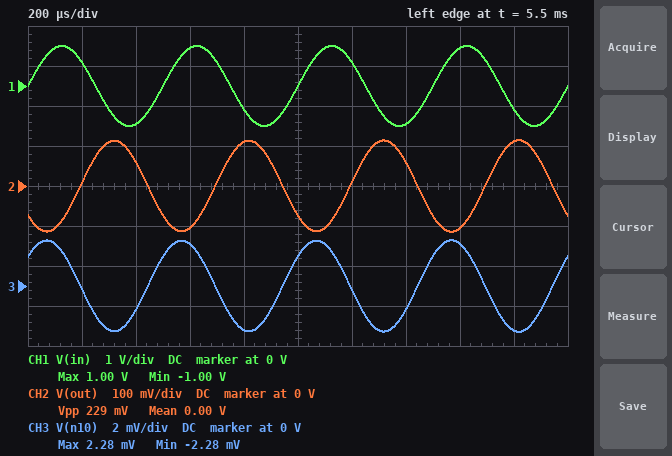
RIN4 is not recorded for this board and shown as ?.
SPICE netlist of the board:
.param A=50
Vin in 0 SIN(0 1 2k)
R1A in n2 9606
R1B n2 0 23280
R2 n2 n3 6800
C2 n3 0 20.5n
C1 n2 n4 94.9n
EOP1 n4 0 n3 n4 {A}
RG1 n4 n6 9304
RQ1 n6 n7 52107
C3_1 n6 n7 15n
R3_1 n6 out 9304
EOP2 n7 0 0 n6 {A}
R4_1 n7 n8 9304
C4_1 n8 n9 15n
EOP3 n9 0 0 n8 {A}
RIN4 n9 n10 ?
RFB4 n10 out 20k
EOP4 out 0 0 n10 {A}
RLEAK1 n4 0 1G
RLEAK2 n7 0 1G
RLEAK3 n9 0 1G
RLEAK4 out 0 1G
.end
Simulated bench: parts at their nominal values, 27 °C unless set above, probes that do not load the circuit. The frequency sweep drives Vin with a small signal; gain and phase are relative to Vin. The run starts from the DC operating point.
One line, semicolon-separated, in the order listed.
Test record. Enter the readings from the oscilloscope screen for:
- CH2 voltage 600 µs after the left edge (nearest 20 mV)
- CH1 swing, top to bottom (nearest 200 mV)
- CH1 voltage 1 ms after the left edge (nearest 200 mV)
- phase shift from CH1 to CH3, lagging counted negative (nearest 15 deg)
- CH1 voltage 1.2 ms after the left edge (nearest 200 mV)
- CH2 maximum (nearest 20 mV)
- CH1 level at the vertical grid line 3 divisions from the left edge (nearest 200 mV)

-100 mV; 2.0 V; 0 V; 45 deg; 600 mV; 120 mV; 1.0 V
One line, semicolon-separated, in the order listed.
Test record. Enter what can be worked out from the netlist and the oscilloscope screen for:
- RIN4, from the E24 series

8.2 kΩ
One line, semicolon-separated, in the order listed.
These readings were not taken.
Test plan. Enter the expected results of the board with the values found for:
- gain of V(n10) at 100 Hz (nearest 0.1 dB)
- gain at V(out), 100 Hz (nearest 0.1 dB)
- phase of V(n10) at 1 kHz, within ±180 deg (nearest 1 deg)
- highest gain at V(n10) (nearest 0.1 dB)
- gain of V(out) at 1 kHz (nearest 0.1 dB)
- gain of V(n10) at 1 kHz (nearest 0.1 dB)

-37.0 dB; -3.0 dB; -153 deg; -35.3 dB; -9.5 dB; -43.5 dB
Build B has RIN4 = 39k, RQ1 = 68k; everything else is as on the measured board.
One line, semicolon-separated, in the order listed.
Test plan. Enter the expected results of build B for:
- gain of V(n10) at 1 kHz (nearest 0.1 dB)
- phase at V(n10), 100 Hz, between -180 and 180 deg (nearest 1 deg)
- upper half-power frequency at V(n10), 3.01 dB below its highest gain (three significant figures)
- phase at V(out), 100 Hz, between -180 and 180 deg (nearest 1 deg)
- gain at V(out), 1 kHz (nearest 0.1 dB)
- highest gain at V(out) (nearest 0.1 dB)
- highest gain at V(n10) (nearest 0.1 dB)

-44.0 dB; -13 deg; 836 Hz; 167 deg; -10.0 dB; 3.1 dB; -30.9 dB
